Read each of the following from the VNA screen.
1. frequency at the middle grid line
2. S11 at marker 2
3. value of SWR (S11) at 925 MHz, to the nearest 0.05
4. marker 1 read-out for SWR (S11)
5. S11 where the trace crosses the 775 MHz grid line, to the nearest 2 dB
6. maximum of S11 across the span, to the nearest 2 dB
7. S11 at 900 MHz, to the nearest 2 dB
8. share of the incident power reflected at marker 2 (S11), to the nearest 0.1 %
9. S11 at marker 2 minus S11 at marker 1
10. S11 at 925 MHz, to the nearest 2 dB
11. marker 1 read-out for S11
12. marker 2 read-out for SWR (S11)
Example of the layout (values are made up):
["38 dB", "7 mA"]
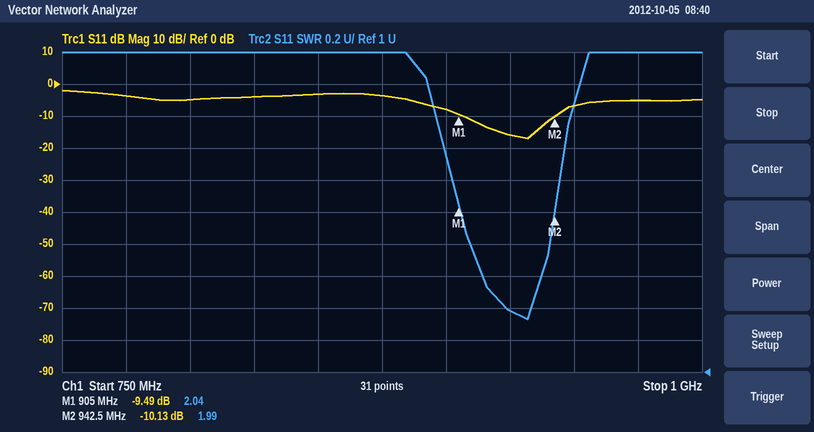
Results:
["875 MHz", "-10.13 dB", "1.40", "2.04", "-4 dB", "-2 dB", "-8 dB", "9.7 %", "-0.64 dB", "-16 dB", "-9.49 dB", "1.99"]
